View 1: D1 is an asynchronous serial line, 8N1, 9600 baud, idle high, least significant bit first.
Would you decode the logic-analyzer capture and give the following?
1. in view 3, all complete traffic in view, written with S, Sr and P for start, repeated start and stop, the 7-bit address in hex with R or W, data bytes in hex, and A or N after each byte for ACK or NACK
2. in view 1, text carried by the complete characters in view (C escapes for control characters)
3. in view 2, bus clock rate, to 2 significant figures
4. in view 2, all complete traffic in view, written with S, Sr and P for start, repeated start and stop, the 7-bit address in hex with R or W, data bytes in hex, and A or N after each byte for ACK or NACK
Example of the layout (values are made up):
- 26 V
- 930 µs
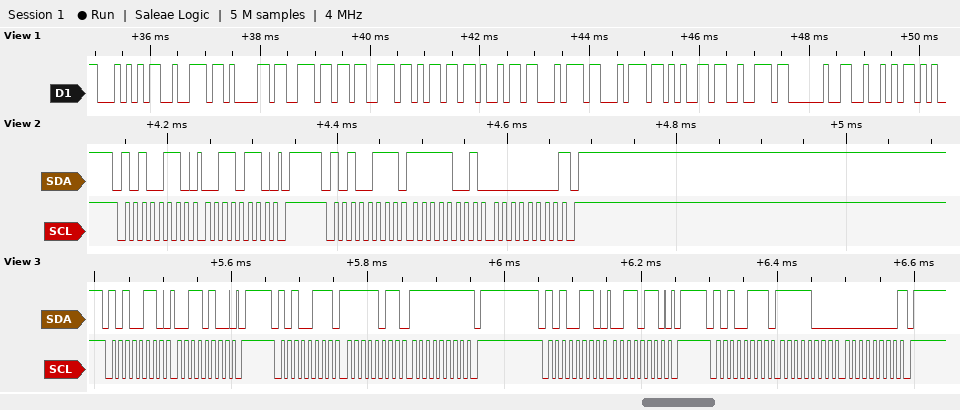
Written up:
- S 53W A 34 A P S 53R A FB A FF N P S 53W A 36 A P S 53R A F8 A 00 N P
- "Transmitter R"
- 100 kHz
- S 53W A 36 A P S 53R A F9 A 00 N P
